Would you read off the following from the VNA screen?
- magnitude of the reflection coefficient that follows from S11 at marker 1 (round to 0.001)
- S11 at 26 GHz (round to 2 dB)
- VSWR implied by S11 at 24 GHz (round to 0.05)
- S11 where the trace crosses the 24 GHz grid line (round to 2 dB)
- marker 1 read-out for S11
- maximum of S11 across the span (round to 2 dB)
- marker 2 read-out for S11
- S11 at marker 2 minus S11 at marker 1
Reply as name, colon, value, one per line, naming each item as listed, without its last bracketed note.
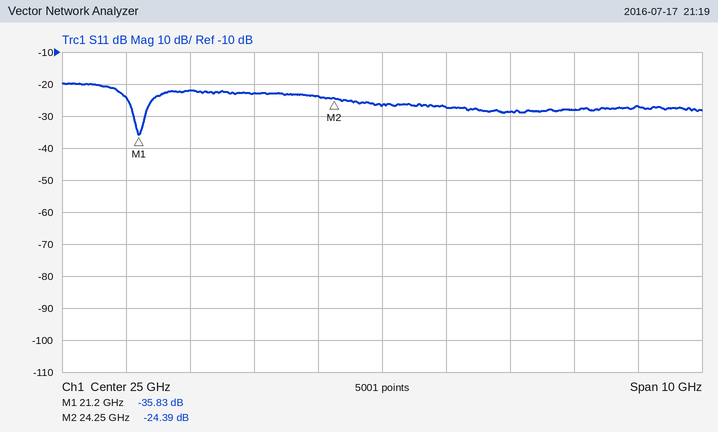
magnitude of the reflection coefficient that follows from S11 at marker 1: 0.016
S11 at 26 GHz: -28 dB
VSWR implied by S11 at 24 GHz: 1.15
S11 where the trace crosses the 24 GHz grid line: -24 dB
marker 1 read-out for S11: -35.83 dB
maximum of S11 across the span: -20 dB
marker 2 read-out for S11: -24.39 dB
S11 at marker 2 minus S11 at marker 1: 11.44 dB
